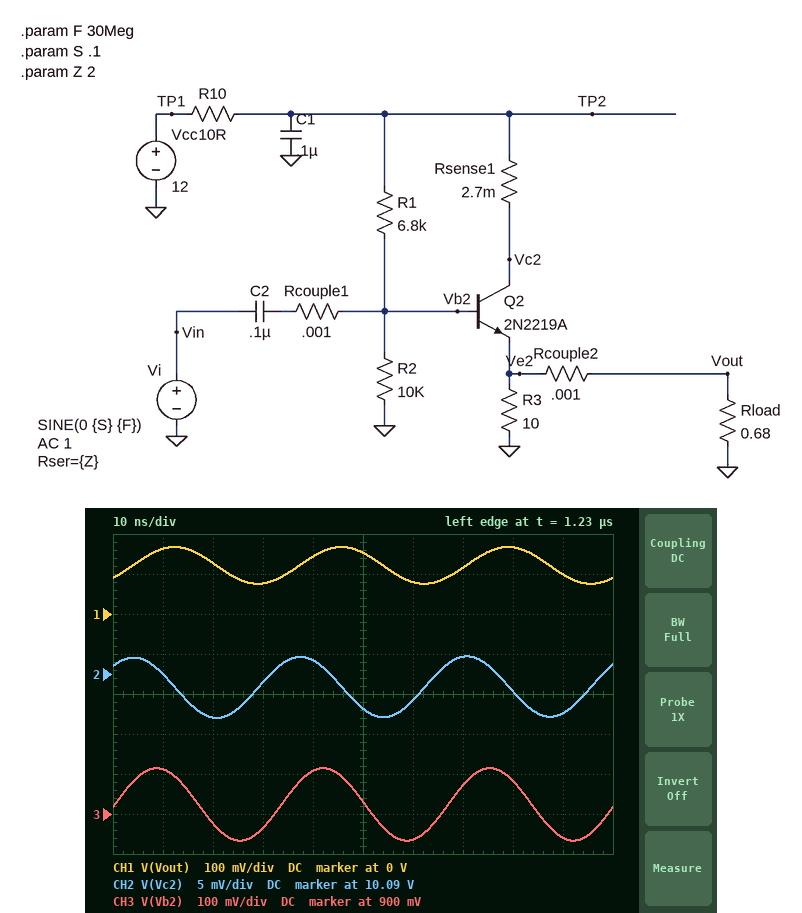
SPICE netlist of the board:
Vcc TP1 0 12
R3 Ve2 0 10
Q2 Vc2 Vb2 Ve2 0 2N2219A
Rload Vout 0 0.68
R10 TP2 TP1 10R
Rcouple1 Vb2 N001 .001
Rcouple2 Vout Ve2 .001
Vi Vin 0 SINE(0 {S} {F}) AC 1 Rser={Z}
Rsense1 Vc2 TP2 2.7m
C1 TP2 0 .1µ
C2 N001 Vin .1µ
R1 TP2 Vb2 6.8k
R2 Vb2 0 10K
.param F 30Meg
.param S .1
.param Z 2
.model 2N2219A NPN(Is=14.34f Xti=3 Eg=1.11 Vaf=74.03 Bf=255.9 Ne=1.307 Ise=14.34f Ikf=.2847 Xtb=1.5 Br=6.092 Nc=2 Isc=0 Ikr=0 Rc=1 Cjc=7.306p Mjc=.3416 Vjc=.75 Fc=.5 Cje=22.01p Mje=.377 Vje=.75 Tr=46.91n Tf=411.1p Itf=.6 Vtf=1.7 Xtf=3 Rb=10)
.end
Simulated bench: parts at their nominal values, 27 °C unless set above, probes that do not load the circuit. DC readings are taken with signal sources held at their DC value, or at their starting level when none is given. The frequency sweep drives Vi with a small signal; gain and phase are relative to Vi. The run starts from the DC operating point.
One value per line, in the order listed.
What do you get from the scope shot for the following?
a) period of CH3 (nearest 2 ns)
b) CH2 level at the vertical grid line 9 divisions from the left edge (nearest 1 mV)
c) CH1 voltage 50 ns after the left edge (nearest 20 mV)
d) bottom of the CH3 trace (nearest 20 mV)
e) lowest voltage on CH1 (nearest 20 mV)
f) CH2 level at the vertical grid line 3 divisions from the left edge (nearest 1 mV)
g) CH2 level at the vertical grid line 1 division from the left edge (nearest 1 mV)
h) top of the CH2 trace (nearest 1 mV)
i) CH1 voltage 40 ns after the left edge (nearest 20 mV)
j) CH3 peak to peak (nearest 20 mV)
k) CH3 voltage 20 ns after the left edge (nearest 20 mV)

34 ns
10.085 V
160 mV
840 mV
80 mV
10.089 V
10.090 V
10.092 V
140 mV
180 mV
880 mV
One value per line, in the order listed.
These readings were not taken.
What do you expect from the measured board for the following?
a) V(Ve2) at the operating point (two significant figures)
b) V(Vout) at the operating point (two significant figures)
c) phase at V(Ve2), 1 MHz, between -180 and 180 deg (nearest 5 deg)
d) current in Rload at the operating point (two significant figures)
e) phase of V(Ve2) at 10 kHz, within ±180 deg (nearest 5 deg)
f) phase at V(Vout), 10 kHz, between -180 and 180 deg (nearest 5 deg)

120 mV
120 mV
0 deg
180 mA
60 deg
60 deg
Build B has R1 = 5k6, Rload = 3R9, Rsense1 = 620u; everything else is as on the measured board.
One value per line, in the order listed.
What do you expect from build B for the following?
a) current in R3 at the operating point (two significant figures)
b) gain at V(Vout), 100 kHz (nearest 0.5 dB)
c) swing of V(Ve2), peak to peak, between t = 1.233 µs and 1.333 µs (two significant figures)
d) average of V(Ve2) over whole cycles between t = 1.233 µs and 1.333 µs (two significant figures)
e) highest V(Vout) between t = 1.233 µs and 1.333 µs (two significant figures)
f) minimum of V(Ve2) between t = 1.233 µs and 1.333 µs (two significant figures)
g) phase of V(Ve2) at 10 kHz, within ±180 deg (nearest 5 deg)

57 mA
-1.0 dB
170 mV
570 mV
660 mV
490 mV
30 deg
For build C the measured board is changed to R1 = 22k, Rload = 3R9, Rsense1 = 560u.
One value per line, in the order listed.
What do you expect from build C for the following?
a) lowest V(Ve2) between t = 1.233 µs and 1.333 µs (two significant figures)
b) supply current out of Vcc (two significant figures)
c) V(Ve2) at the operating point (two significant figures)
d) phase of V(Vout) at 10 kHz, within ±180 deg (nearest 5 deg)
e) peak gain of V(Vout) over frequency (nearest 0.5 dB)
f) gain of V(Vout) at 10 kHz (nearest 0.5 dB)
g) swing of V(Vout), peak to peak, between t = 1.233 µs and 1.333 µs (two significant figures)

120 mV
71 mA
200 mV
20 deg
-1.5 dB
-2.0 dB
160 mV
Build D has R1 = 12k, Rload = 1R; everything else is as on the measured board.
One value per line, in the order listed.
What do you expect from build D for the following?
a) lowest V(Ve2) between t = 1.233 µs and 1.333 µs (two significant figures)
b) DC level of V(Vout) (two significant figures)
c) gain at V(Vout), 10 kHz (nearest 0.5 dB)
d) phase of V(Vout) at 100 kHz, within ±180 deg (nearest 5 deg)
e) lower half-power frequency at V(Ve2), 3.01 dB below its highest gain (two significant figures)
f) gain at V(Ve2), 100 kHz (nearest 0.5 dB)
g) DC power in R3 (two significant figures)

60 mV
110 mV
-6.0 dB
5 deg
10 kHz
-3.0 dB
1.3 mW
